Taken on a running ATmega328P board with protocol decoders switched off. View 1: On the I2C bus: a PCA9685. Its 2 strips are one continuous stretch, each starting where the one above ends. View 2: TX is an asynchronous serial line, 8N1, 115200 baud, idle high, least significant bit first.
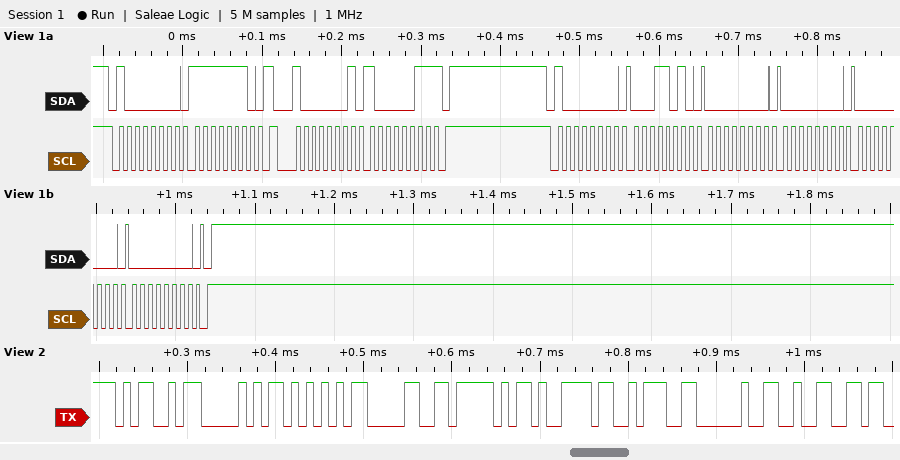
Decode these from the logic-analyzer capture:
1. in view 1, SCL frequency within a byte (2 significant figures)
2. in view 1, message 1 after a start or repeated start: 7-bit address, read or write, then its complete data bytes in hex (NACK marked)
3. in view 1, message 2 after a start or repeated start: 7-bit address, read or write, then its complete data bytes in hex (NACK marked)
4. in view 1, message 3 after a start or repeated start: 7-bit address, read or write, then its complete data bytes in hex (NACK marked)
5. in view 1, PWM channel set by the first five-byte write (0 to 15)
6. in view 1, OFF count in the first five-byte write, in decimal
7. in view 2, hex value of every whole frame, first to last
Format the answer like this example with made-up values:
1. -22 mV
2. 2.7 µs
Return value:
1. 100 kHz
2. 0x40 write: FE
3. 0x40 read: 83 NACK
4. 0x40 write: 1A 00 00 00 00
5. 5
6. 0
7. 4D 50 55 30 5F 79 3A 20 32
